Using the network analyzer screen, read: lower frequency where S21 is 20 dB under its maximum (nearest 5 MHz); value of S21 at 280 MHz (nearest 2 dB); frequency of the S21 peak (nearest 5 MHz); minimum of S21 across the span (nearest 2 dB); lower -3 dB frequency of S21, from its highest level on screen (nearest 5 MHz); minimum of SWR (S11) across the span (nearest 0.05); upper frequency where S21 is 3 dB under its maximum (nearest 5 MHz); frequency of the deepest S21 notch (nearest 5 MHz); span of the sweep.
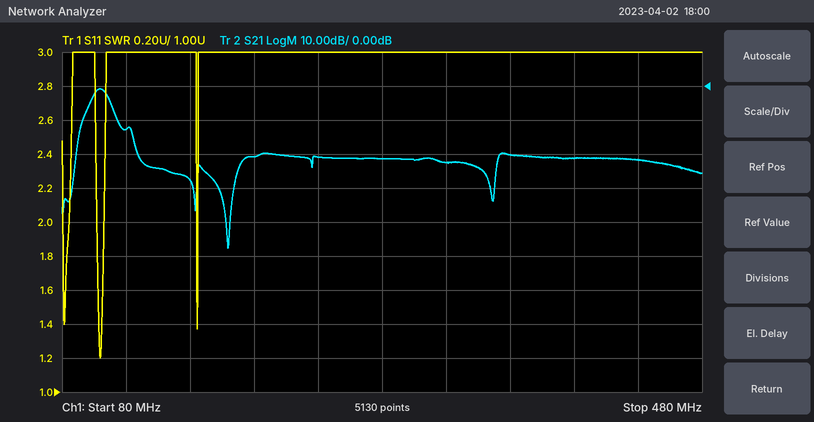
90 MHz
-22 dB
105 MHz
-48 dB
100 MHz
1.20
110 MHz
185 MHz
400 MHz
